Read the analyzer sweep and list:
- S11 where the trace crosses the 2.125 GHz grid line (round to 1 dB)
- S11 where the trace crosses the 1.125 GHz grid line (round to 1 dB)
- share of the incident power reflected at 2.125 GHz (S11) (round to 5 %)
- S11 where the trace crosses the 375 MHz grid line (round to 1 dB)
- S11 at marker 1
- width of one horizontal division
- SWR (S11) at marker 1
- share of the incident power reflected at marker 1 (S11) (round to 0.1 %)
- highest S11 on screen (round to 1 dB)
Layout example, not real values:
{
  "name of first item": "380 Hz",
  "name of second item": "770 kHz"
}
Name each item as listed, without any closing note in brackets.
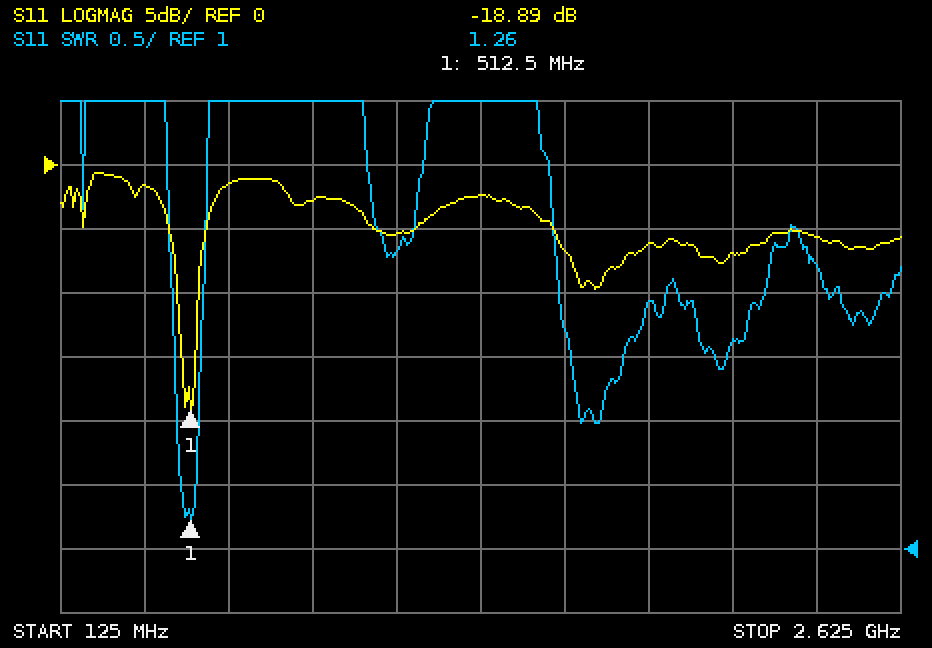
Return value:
{
  "S11 where the trace crosses the 2.125 GHz grid line": "-7 dB",
  "S11 where the trace crosses the 1.125 GHz grid line": "-5 dB",
  "share of the incident power reflected at 2.125 GHz (S11)": "20 %",
  "S11 where the trace crosses the 375 MHz grid line": "-2 dB",
  "S11 at marker 1": "-18.89 dB",
  "width of one horizontal division": "250 MHz",
  "SWR (S11) at marker 1": "1.26",
  "share of the incident power reflected at marker 1 (S11)": "1.3 %",
  "highest S11 on screen": "-1 dB"
}
